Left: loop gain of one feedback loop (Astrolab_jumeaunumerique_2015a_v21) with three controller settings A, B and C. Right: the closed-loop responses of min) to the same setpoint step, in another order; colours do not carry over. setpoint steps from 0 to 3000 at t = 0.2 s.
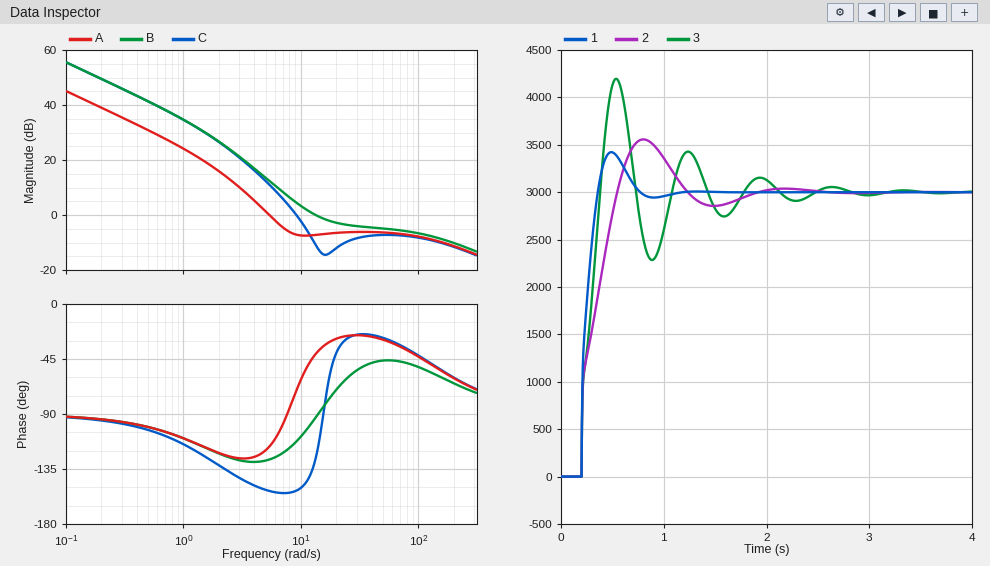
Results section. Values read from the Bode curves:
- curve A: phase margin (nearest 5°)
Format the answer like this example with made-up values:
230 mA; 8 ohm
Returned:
65°
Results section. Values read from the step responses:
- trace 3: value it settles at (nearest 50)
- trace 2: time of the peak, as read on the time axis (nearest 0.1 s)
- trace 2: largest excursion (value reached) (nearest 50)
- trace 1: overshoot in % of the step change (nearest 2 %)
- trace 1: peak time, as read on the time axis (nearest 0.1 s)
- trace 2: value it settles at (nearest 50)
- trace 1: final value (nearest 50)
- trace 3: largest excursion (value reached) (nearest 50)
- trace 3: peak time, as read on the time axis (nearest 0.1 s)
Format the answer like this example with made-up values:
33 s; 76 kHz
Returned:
3000; 0.8 s; 3550; 14 %; 0.5 s; 3000; 3000; 4200; 0.5 s
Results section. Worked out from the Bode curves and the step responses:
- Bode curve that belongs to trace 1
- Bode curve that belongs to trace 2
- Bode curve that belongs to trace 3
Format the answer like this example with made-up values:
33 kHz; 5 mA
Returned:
B; A; C
